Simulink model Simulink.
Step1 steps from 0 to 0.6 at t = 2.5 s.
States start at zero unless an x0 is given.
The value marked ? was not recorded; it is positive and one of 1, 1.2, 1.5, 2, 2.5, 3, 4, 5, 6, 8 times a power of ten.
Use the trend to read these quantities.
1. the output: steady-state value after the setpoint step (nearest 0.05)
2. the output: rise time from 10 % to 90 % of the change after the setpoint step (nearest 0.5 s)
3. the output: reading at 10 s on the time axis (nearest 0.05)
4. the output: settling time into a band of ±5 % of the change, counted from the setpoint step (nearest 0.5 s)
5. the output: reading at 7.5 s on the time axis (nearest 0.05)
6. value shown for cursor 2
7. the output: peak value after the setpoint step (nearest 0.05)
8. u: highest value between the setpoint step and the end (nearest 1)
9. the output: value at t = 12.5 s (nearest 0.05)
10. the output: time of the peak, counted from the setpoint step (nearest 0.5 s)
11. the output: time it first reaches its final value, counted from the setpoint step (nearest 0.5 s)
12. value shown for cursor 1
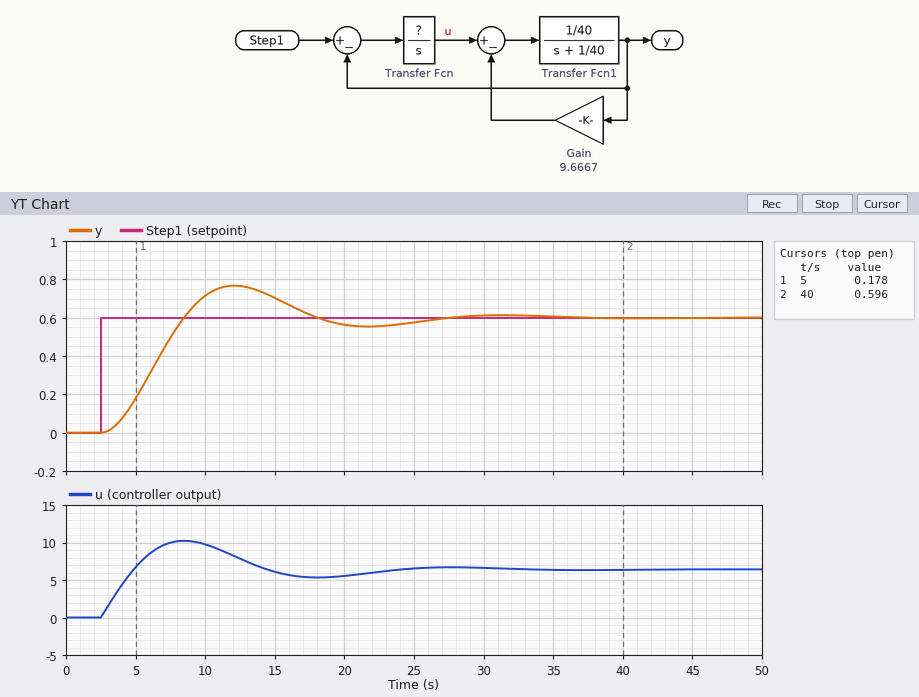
0.60
4.0 s
0.70
22.0 s
0.50
0.596
0.75
10
0.75
9.5 s
6.0 s
0.178
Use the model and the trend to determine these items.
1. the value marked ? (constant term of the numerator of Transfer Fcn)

5
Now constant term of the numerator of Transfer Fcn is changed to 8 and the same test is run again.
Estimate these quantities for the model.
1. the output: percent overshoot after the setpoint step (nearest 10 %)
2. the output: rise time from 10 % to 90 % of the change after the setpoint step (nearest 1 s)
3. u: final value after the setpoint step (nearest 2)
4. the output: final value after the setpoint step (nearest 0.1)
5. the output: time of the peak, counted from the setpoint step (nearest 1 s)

40 %
3 s
6
0.6
7 s
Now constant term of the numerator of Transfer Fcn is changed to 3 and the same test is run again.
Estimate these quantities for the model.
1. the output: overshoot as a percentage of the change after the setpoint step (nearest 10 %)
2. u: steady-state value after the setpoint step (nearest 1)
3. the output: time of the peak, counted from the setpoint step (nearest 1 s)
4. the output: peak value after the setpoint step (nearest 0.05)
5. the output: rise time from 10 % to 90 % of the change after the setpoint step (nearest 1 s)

20 %
6
13 s
0.70
6 s
